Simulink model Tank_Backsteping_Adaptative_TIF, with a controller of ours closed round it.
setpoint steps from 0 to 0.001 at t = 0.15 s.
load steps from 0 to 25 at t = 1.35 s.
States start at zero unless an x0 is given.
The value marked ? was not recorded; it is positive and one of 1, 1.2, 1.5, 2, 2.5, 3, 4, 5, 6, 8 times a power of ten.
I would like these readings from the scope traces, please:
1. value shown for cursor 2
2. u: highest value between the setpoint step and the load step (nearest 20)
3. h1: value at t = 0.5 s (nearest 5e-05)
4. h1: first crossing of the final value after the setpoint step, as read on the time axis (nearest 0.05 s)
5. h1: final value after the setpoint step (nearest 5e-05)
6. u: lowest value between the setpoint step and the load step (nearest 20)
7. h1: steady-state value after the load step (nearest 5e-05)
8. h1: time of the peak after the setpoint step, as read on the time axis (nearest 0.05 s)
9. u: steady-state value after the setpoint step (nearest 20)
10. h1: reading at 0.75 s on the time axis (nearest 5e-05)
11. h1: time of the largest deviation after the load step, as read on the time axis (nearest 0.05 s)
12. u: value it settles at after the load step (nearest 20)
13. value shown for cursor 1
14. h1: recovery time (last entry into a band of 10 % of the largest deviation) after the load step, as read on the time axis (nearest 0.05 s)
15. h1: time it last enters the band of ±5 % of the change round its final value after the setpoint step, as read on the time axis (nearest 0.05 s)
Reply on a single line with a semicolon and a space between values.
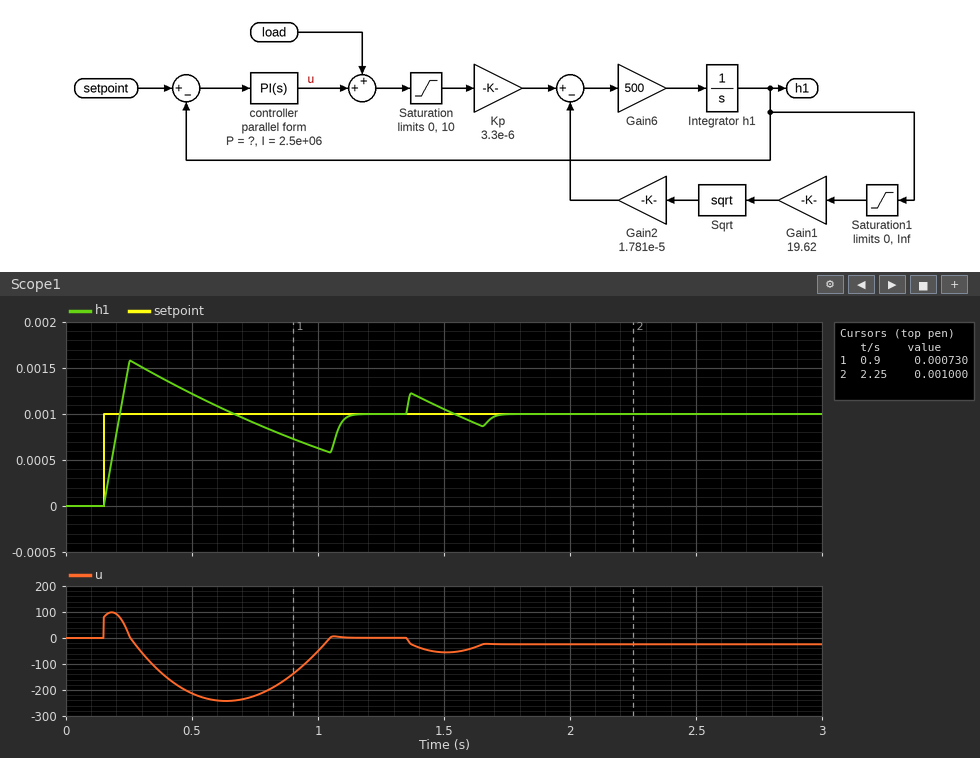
0.001000; 100; 0.00120; 0.20 s; 0.00100; -240; 0.00100; 0.25 s; 0; 0.00090; 1.35 s; -20; 0.000730; 1.70 s; 1.10 s
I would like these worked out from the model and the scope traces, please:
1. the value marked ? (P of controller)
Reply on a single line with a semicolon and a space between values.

80000
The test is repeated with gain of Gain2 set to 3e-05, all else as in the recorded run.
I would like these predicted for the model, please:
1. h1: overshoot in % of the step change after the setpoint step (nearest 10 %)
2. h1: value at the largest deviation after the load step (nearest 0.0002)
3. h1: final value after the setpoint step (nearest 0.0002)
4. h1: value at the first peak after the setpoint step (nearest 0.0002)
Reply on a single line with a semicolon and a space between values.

60 %; 0.0012; 0.0010; 0.0016
